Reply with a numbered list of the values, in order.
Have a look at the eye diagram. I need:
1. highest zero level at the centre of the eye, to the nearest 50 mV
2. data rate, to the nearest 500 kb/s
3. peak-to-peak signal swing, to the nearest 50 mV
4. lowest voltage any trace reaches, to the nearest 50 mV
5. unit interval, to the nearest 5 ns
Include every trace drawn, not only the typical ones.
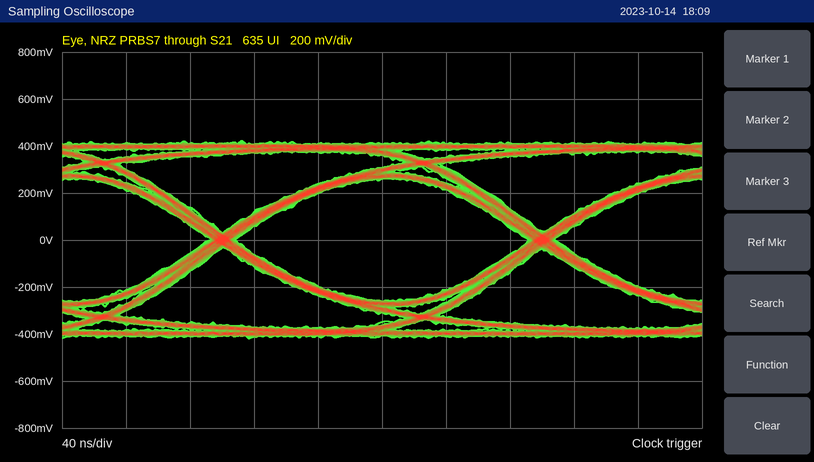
1. -250 mV
2. 5.0 Mb/s
3. 850 mV
4. -400 mV
5. 200 ns
